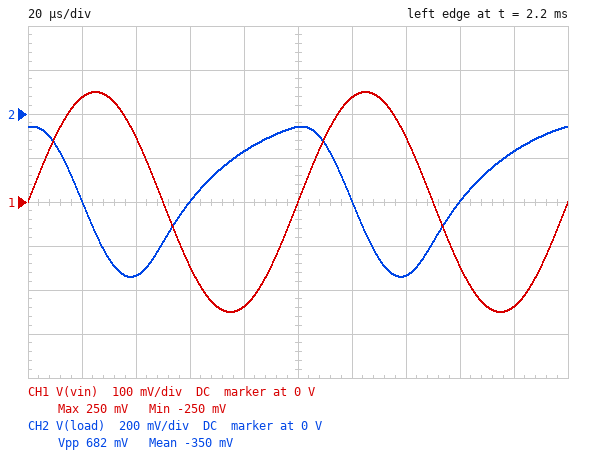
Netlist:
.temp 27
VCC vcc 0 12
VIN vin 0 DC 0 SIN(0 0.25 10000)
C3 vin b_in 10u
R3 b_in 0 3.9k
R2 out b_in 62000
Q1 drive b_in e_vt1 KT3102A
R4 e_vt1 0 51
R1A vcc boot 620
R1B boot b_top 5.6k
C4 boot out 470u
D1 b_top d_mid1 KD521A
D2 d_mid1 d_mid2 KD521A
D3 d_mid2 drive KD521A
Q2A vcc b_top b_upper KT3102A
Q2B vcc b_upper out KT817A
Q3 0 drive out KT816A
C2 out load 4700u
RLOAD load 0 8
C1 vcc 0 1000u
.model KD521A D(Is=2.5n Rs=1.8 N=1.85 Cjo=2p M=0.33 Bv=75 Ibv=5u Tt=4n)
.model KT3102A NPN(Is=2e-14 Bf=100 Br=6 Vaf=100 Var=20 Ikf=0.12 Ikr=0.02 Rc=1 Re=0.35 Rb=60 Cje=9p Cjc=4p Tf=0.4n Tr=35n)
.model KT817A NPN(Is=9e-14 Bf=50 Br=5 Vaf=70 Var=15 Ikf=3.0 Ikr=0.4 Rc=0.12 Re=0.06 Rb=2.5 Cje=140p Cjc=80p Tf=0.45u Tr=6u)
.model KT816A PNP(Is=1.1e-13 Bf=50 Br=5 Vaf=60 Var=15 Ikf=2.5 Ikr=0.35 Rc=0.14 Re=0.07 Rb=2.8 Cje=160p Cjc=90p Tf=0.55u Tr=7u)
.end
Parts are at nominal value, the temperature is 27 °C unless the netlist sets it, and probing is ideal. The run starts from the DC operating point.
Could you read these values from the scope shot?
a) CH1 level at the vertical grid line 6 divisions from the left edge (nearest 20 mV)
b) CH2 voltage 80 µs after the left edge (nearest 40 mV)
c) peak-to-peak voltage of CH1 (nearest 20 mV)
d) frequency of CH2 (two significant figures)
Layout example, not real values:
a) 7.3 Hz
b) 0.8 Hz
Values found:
a) 240 mV
b) -160 mV
c) 500 mV
d) 10 kHz
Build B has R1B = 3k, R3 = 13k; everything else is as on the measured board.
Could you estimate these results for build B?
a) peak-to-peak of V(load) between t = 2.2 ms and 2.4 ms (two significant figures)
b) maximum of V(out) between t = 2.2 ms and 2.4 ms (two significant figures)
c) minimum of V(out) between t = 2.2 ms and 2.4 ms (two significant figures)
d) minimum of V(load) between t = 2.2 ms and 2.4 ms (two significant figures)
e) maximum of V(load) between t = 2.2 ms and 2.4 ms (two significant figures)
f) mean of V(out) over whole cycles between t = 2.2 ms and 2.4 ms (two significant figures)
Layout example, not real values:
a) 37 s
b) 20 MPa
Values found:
a) 6.1 V
b) 11 V
c) 5.0 V
d) -450 mV
e) 5.6 V
f) 7.1 V
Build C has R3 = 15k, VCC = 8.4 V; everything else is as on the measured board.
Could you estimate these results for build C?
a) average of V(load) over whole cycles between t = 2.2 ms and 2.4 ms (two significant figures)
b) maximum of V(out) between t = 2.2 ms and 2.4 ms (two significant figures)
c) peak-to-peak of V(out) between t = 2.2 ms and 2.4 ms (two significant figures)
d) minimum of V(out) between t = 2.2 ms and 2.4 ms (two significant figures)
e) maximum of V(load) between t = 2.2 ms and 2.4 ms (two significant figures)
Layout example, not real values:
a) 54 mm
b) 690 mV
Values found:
a) 580 mV
b) 7.4 V
c) 4.0 V
d) 3.4 V
e) 3.6 V
